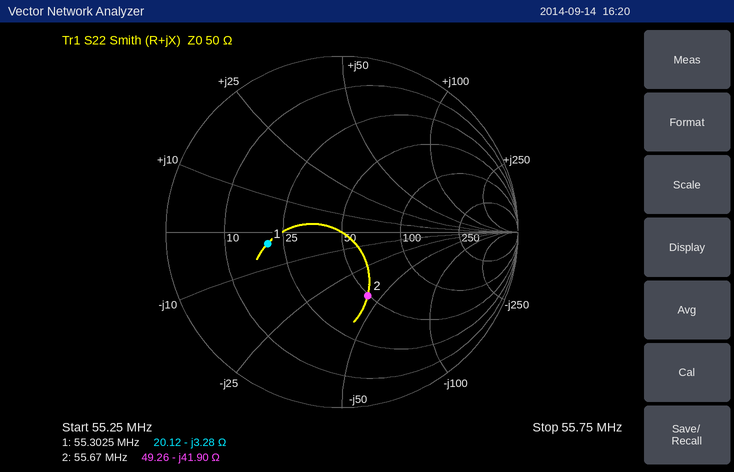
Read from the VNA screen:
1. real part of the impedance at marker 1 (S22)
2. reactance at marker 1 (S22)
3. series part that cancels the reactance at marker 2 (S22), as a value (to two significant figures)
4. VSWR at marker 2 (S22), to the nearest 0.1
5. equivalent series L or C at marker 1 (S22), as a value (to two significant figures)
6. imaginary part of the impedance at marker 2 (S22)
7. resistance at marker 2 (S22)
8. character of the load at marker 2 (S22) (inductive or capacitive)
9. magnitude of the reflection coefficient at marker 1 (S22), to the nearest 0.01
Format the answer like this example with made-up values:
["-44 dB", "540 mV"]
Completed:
["20.12 Ω", "-3.28 Ω", "120 nH", "2.3", "880 pF", "-41.90 Ω", "49.26 Ω", "capacitive", "0.43"]
